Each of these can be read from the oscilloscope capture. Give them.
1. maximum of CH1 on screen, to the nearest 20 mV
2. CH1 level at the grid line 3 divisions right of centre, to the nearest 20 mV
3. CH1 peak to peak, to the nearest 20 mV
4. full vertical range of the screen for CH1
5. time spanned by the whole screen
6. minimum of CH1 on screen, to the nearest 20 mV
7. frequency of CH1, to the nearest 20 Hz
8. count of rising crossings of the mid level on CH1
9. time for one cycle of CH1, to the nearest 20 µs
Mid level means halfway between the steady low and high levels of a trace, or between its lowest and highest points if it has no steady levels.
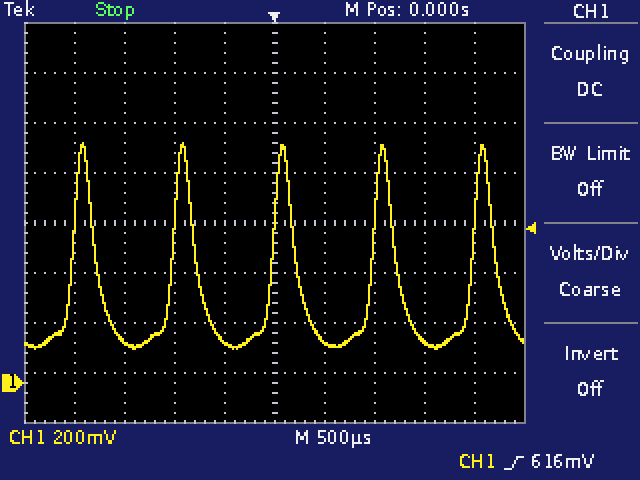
960 mV
160 mV
820 mV
1.6 V
5 ms
140 mV
1.00 kHz
5
1.00 ms
